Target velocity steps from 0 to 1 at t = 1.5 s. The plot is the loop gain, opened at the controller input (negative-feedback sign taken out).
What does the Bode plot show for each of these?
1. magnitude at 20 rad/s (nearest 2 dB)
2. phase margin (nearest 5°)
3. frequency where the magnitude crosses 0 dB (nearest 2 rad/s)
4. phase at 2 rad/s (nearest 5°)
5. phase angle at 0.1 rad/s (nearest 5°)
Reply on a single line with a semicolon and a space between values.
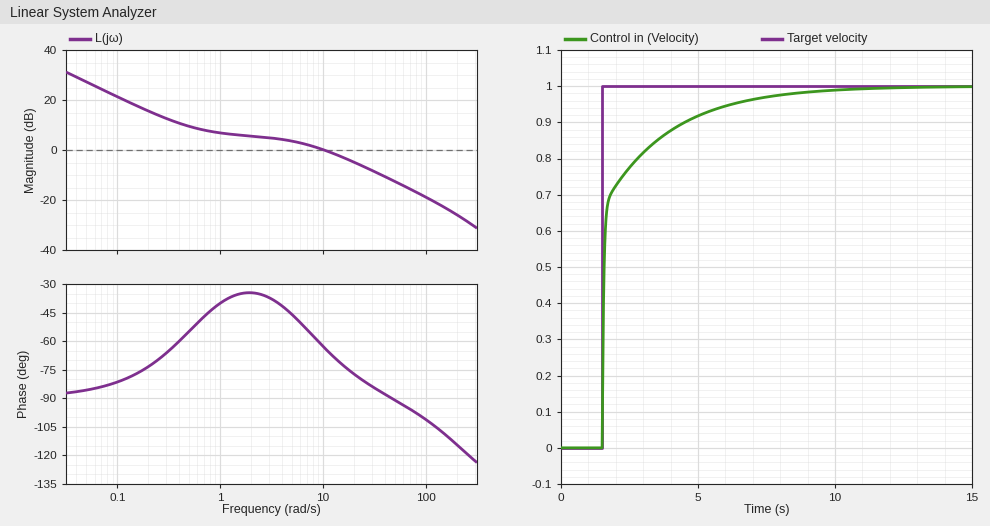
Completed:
-4 dB; 115°; 10 rad/s; -35°; -80°
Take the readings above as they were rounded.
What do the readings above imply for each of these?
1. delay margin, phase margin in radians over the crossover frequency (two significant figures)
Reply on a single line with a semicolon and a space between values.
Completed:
0.20 s
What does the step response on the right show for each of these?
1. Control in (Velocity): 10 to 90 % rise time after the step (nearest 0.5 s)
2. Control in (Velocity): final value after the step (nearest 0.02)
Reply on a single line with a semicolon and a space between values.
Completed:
3.0 s; 1.00
